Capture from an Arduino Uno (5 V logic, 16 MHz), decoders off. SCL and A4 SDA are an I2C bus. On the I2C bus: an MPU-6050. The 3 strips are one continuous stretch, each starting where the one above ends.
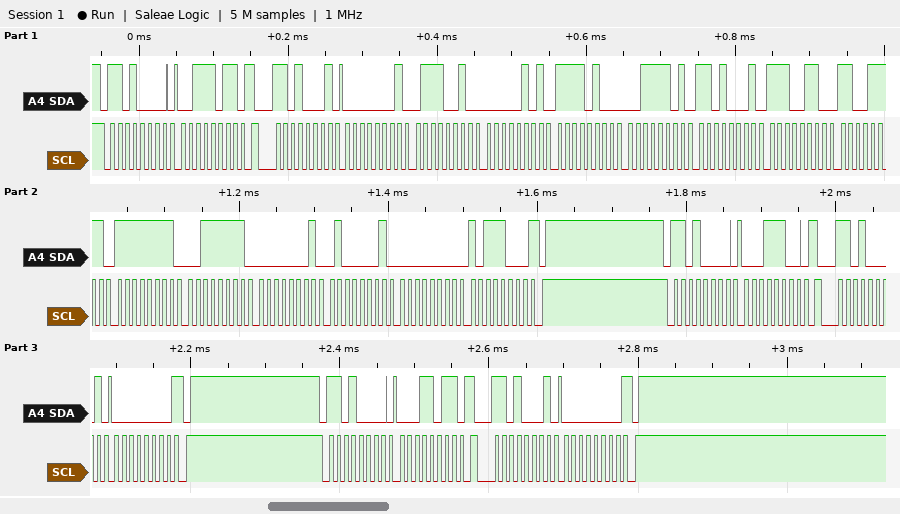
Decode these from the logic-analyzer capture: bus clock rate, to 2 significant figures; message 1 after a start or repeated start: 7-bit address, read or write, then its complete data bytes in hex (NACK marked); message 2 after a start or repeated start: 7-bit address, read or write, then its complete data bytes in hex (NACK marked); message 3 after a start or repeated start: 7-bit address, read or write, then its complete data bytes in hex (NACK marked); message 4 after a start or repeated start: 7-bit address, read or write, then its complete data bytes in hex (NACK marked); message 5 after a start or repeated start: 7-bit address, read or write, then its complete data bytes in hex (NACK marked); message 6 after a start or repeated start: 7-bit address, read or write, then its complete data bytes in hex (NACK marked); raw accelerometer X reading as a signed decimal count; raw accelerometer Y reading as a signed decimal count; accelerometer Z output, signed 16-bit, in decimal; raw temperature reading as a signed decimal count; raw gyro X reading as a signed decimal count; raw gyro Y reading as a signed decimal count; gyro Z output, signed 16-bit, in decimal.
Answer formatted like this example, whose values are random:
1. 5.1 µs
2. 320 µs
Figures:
1. 100 kHz
2. 0x68 write: 3B
3. 0x68 read: 01 72 05 F4 3D D1 E6 CF FF 3F 01 41 00 B8 NACK
4. 0x68 write: 1C
5. 0x68 read: 00 NACK
6. 0x68 write: 1B
7. 0x68 read: 00 NACK
8. 370
9. 1524
10. 15825
11. -6449
12. -193
13. 321
14. 184
